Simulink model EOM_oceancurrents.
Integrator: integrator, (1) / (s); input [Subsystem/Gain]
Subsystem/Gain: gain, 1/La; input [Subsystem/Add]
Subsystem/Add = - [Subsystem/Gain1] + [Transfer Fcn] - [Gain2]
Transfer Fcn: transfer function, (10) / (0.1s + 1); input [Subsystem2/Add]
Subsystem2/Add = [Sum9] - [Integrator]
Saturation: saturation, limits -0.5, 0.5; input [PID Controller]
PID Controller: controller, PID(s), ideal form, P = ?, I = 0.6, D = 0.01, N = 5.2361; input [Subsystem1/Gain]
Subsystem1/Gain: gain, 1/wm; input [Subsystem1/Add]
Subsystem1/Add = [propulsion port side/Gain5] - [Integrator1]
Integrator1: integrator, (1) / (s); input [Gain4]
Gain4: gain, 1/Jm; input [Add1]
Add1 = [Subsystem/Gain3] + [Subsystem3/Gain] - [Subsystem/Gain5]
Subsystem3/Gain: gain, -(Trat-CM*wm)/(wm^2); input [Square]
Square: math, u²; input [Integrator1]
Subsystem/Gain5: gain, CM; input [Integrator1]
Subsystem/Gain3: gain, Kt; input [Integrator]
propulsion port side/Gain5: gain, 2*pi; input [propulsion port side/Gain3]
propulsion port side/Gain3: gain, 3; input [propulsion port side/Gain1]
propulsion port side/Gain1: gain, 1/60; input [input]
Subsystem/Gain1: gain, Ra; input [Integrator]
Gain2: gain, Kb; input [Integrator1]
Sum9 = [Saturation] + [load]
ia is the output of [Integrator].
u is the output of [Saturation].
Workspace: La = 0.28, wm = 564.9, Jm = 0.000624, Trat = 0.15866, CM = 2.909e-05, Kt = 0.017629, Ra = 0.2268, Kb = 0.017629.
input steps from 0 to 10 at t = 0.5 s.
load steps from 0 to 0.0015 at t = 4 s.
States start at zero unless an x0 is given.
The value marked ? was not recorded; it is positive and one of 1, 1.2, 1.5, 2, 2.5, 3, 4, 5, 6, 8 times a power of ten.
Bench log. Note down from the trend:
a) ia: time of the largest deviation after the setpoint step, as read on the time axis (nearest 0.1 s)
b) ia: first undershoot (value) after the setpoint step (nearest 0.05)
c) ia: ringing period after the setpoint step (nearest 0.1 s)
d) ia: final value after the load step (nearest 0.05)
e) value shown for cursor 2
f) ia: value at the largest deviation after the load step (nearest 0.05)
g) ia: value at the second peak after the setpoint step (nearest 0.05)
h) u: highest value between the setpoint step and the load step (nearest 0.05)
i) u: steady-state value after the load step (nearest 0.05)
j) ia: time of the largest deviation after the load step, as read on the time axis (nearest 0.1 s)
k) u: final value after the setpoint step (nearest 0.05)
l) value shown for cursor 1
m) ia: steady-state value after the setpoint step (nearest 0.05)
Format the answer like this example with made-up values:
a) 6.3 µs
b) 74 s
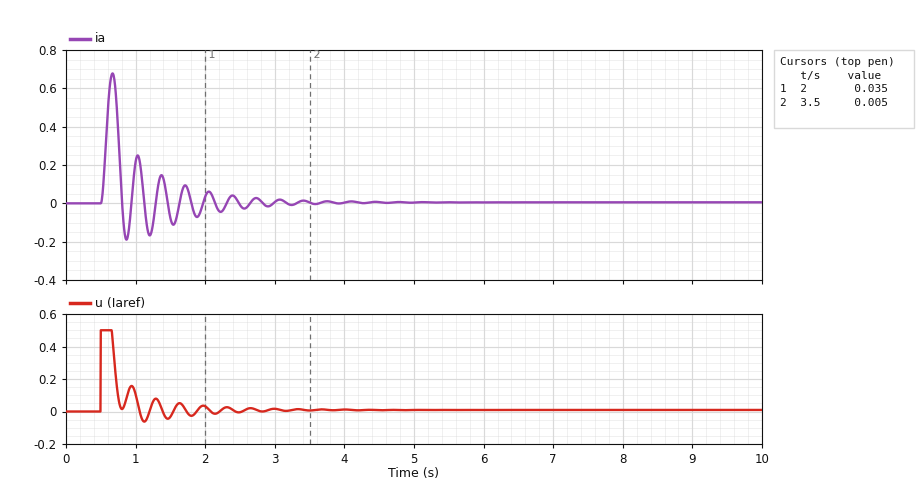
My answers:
a) 0.7 s
b) -0.20
c) 0.4 s
d) 0.00
e) 0.005
f) 0.00
g) 0.25
h) 0.50
i) 0.00
j) 4.1 s
k) 0.00
l) 0.035
m) 0.00
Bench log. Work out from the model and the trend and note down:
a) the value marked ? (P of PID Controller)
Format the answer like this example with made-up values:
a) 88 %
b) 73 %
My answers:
a) 150
